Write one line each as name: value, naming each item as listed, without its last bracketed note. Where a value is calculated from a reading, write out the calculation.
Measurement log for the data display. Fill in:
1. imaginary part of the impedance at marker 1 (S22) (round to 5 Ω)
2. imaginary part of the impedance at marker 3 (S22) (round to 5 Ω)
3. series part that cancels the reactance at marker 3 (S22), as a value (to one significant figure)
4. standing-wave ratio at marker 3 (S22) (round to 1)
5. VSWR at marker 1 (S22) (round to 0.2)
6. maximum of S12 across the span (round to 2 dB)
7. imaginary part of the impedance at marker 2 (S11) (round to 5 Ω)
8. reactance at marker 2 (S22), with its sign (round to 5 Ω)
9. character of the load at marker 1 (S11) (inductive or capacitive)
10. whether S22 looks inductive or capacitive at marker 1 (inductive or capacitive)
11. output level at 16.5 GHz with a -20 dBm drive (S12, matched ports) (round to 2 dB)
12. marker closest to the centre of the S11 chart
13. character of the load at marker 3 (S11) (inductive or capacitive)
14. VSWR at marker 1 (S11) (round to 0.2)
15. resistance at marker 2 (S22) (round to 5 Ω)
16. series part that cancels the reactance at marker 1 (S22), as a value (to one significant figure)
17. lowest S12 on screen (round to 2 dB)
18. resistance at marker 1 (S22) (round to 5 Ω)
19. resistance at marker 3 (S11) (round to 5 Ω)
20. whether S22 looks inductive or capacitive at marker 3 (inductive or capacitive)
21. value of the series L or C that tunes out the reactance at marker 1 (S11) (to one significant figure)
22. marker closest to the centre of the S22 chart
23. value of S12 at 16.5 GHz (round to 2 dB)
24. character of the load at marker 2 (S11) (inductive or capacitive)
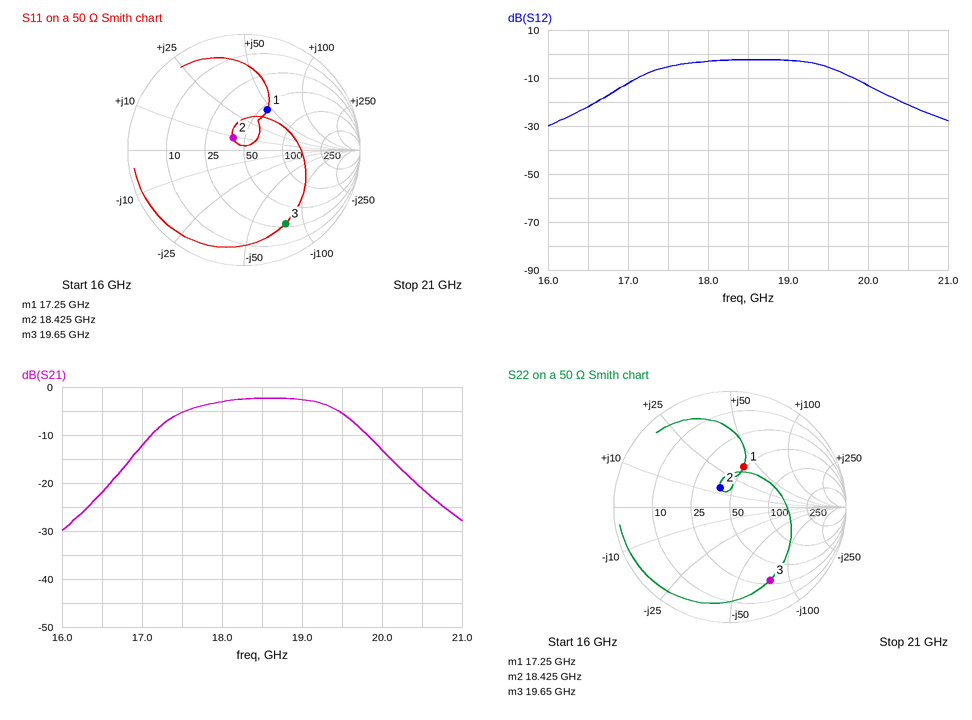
imaginary part of the impedance at marker 1 (S22): +40 Ω
imaginary part of the impedance at marker 3 (S22): -75 Ω
series part that cancels the reactance at marker 3 (S22), as a value: L = 75 Ω/(2π × 19.65 GHz) ≈ 607 pH, so 600 pH to one significant figure
standing-wave ratio at marker 3 (S22): 6
VSWR at marker 1 (S22): 2.2
maximum of S12 across the span: -2 dB
imaginary part of the impedance at marker 2 (S11): +10 Ω
reactance at marker 2 (S22), with its sign: +15 Ω
character of the load at marker 1 (S11): inductive
whether S22 looks inductive or capacitive at marker 1: inductive
output level at 16.5 GHz with a -20 dBm drive (S12, matched ports): -20 dBm + (-22 dB) = -42 dBm
marker closest to the centre of the S11 chart: marker 2
character of the load at marker 3 (S11): capacitive
VSWR at marker 1 (S11): 2.4
resistance at marker 2 (S22): 40 Ω
series part that cancels the reactance at marker 1 (S22), as a value: C = 1/(2π × 17.25 GHz × 40 Ω) ≈ 231 fF, so 200 fF to one significant figure
lowest S12 on screen: -30 dB
resistance at marker 1 (S22): 50 Ω
resistance at marker 3 (S11): 30 Ω
whether S22 looks inductive or capacitive at marker 3: capacitive
value of the series L or C that tunes out the reactance at marker 1 (S11): C = 1/(2π × 17.25 GHz × 45 Ω) ≈ 205 fF, so 200 fF to one significant figure
marker closest to the centre of the S22 chart: marker 2
value of S12 at 16.5 GHz: -22 dB
character of the load at marker 2 (S11): inductive
